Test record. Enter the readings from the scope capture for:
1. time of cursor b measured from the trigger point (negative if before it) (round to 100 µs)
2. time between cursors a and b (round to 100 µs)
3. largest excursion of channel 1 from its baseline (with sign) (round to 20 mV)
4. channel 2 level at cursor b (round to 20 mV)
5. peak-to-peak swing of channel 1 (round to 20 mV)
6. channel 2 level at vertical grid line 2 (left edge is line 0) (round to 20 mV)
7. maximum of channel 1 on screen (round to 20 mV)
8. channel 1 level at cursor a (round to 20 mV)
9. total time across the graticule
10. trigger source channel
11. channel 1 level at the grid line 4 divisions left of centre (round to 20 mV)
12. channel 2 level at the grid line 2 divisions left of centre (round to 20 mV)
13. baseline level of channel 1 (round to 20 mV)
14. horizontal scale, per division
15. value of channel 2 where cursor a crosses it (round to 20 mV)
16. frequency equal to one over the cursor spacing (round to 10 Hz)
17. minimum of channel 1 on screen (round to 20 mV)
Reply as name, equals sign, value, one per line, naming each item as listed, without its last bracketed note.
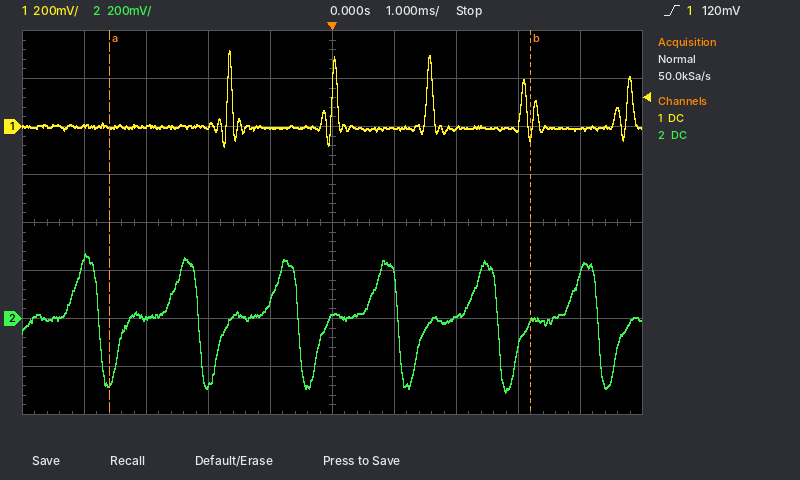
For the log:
time of cursor b measured from the trigger point (negative if before it) = +3.2 ms
time between cursors a and b = 6.8 ms
largest excursion of channel 1 from its baseline (with sign) = +320 mV
channel 2 level at cursor b = -20 mV
peak-to-peak swing of channel 1 = 400 mV
channel 2 level at vertical grid line 2 (left edge is line 0) = 0 mV
maximum of channel 1 on screen = 320 mV
channel 1 level at cursor a = 0 mV
total time across the graticule = 10 ms
trigger source channel = channel 1
channel 1 level at the grid line 4 divisions left of centre = 0 mV
channel 2 level at the grid line 2 divisions left of centre = -280 mV
baseline level of channel 1 = 0 mV
horizontal scale, per division = 1 ms
value of channel 2 where cursor a crosses it = -260 mV
frequency equal to one over the cursor spacing = 150 Hz
minimum of channel 1 on screen = -80 mV
